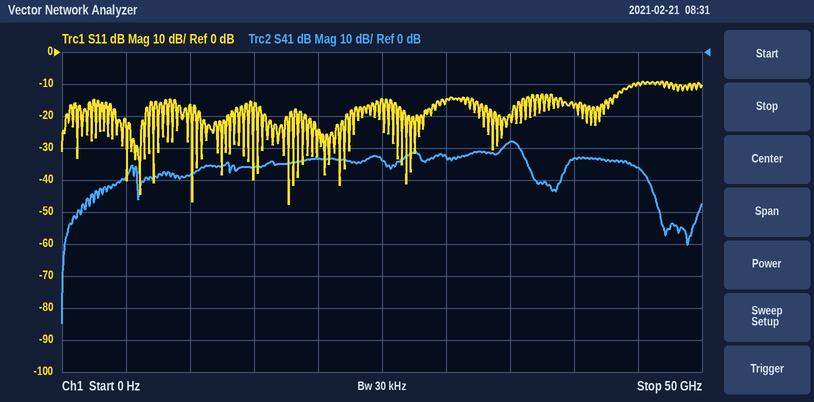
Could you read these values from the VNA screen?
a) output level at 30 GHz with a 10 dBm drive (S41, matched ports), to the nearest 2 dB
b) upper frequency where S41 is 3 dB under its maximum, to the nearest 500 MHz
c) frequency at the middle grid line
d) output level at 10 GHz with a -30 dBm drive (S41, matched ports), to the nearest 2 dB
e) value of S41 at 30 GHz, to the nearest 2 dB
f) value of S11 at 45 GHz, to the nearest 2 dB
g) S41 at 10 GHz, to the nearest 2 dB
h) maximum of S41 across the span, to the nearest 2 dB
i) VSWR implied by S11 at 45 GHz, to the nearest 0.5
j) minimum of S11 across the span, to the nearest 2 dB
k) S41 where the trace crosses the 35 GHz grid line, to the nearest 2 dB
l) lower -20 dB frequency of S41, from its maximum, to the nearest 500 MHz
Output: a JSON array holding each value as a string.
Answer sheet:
["-22 dBm", "36.0 GHz", "25 GHz", "-68 dBm", "-32 dB", "-10 dB", "-38 dB", "-28 dB", "2.0", "-48 dB", "-28 dB", "2.0 GHz"]
